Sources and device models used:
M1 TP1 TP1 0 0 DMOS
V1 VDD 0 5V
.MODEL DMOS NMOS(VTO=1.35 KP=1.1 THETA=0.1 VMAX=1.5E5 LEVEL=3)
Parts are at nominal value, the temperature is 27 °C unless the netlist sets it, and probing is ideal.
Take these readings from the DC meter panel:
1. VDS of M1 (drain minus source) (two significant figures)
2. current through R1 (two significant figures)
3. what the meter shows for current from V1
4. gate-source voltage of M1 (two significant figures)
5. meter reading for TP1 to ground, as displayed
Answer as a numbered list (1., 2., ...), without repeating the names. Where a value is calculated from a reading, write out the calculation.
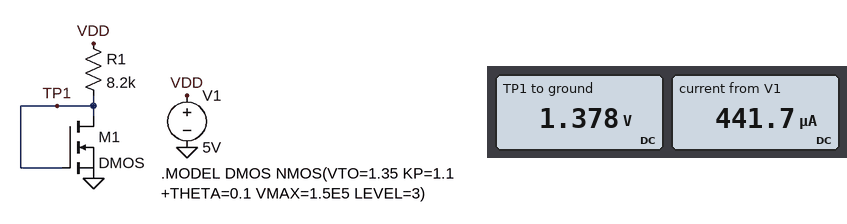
1. 1.378 V = 1.4 V
2. (5 V - 1.378 V) / 8.2 kΩ = 440 µA
3. 441.7 µA
4. 1.378 V = 1.4 V
5. 1.378 V
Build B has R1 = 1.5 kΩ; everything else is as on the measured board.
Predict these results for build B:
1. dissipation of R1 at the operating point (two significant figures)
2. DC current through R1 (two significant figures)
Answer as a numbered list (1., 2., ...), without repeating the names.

1. 8.6 mW
2. 2.4 mA
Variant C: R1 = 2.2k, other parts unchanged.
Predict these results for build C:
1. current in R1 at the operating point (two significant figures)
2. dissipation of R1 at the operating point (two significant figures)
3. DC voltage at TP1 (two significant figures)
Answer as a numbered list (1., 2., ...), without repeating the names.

1. 1.6 mA
2. 5.9 mW
3. 1.4 V
